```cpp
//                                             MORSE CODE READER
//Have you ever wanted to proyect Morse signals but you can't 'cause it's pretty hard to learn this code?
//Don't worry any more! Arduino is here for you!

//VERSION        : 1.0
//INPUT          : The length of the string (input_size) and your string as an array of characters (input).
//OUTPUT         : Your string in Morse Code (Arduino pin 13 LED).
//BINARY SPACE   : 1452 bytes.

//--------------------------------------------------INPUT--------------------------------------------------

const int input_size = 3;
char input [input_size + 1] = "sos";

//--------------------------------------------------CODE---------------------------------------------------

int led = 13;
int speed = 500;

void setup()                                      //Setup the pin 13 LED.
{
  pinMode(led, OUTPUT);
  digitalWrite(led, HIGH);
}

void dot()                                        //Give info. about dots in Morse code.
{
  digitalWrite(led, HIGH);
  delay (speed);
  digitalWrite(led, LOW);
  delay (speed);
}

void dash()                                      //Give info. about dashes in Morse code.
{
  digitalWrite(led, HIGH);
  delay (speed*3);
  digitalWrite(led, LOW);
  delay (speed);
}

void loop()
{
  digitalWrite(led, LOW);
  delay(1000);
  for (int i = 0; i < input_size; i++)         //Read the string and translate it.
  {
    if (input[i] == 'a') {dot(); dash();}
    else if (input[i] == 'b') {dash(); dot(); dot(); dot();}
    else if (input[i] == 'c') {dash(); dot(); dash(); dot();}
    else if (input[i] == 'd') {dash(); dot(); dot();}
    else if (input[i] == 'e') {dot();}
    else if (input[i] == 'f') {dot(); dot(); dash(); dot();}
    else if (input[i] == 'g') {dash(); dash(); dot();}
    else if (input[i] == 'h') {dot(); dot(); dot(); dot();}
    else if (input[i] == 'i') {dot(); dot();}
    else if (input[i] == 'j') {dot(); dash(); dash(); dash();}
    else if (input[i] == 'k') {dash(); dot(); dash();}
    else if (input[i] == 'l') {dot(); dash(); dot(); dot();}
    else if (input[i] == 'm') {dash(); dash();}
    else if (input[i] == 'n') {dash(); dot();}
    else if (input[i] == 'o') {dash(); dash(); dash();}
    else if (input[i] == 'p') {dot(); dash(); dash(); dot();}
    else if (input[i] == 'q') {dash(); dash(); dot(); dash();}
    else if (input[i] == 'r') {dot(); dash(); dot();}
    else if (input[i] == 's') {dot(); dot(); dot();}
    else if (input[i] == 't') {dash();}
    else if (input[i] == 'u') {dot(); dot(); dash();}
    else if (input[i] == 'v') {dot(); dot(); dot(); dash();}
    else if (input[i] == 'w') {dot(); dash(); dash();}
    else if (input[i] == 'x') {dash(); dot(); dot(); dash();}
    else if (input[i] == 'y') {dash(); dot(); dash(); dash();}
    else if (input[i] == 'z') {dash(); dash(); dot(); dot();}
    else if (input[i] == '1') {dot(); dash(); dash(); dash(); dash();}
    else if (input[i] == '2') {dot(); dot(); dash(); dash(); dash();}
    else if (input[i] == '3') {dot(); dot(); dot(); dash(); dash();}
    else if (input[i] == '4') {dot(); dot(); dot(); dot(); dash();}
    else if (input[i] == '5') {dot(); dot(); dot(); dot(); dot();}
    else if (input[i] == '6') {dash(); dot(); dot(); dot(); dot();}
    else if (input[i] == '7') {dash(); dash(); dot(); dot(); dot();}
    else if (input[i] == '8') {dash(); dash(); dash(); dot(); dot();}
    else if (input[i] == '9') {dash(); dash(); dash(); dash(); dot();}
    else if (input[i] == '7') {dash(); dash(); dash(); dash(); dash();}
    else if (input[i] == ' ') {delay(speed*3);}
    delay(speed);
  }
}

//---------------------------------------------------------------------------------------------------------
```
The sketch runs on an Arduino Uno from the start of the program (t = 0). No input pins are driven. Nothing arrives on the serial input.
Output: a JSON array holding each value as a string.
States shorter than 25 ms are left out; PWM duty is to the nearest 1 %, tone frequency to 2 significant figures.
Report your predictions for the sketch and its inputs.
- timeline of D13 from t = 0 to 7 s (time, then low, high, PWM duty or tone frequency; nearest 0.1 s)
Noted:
["0 s low; 1 s high; 1.5 s low; 2 s high; 2.5 s low; 3 s high; 3.5 s low; 4.5 s high; 6 s low; 6.5 s high"]
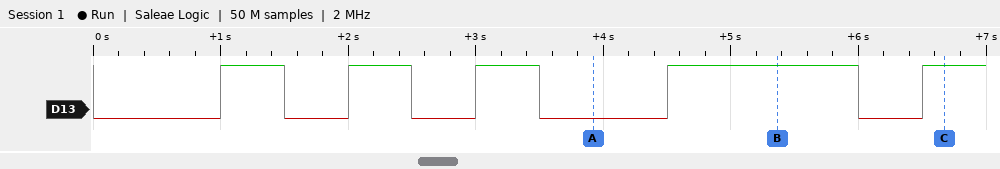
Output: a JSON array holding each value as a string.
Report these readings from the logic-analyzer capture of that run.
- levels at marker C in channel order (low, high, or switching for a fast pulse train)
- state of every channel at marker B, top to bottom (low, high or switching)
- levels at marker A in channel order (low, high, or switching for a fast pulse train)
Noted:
["D13 high", "D13 high", "D13 low"]
